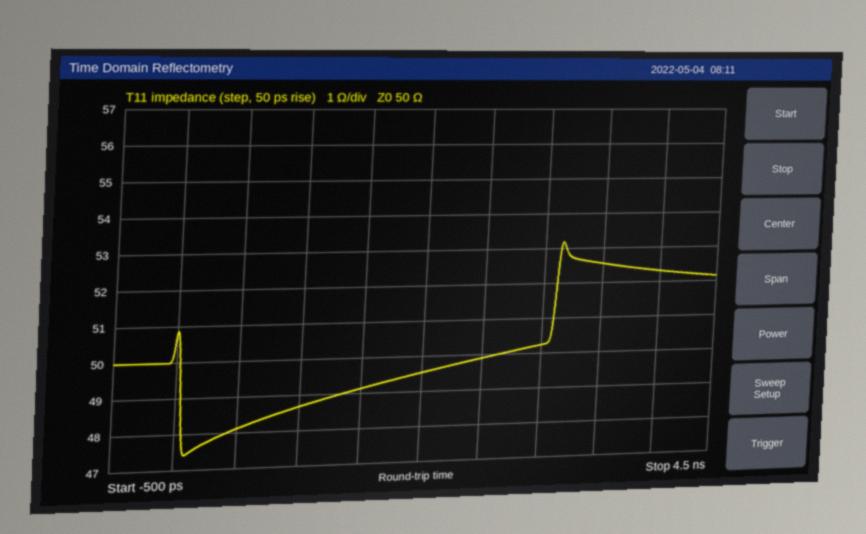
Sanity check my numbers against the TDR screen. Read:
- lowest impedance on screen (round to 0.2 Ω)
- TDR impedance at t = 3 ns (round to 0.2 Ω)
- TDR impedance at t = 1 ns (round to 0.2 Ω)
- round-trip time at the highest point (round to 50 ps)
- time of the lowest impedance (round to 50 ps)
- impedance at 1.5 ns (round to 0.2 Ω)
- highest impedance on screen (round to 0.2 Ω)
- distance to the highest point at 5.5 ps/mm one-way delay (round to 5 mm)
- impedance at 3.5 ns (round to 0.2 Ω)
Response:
47.4 Ω
50.2 Ω
48.6 Ω
3.15 ns
100 ps
49.2 Ω
53.2 Ω
285 mm
52.6 Ω
